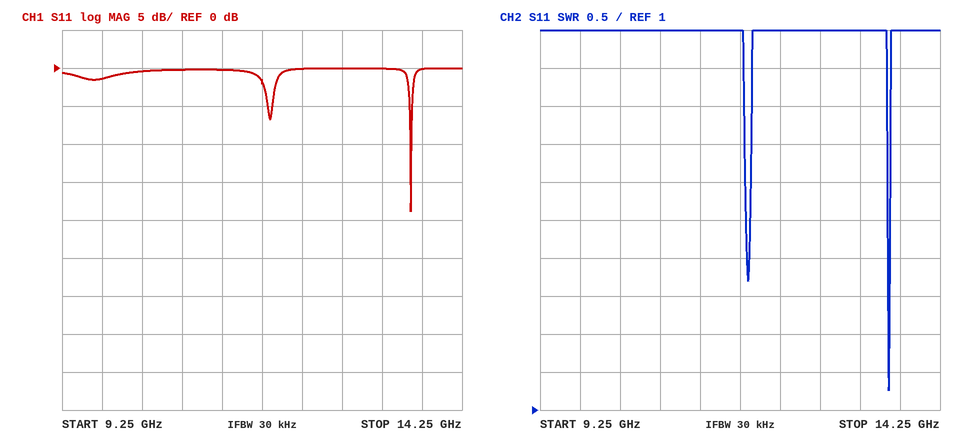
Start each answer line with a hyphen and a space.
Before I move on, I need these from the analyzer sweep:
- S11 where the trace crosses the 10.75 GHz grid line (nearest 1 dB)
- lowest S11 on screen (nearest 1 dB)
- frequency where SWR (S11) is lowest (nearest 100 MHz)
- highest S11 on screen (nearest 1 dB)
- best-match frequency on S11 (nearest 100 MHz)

- 0 dB
- -19 dB
- 13.6 GHz
- 0 dB
- 13.6 GHz
